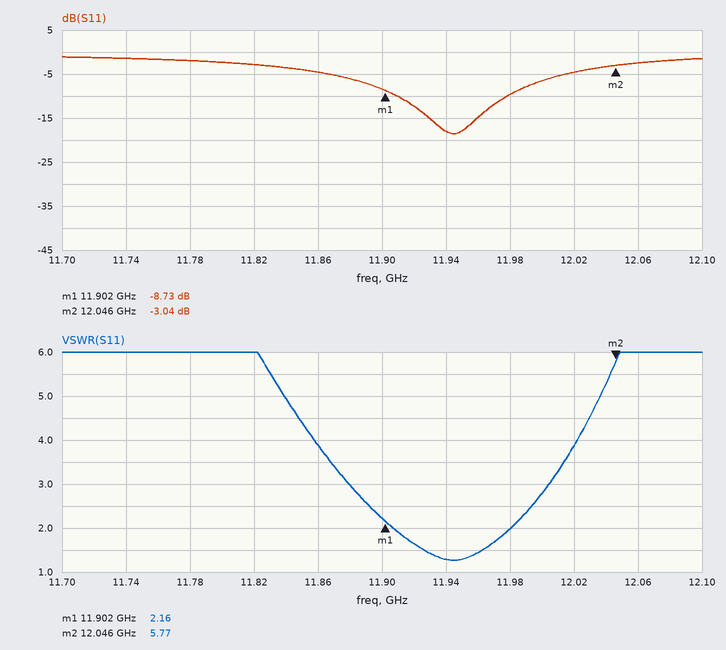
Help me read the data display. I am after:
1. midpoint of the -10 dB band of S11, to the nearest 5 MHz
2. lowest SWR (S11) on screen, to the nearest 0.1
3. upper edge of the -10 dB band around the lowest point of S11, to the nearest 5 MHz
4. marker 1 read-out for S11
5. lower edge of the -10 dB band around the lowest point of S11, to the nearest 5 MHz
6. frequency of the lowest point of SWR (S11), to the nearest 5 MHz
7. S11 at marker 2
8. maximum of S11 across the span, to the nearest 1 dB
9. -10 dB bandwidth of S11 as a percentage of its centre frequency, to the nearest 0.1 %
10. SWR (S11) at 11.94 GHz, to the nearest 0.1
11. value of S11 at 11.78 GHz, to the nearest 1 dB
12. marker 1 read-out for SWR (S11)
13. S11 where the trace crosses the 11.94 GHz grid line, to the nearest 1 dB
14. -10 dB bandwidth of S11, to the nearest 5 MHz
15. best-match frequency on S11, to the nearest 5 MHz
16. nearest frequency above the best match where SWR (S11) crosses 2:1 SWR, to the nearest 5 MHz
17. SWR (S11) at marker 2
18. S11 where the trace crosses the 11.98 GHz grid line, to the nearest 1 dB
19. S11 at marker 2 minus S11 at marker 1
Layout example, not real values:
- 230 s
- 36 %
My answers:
- 11.945 GHz
- 1.3
- 11.980 GHz
- -8.73 dB
- 11.910 GHz
- 11.945 GHz
- -3.04 dB
- -1 dB
- 0.6 %
- 1.3
- -2 dB
- 2.16
- -18 dB
- 70 MHz
- 11.945 GHz
- 11.980 GHz
- 5.77
- -10 dB
- 5.69 dB
